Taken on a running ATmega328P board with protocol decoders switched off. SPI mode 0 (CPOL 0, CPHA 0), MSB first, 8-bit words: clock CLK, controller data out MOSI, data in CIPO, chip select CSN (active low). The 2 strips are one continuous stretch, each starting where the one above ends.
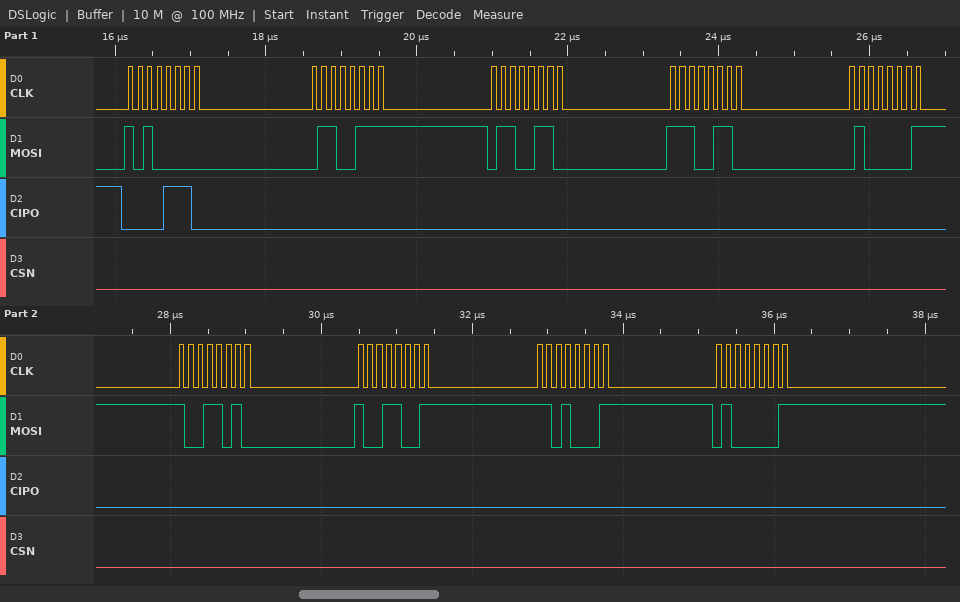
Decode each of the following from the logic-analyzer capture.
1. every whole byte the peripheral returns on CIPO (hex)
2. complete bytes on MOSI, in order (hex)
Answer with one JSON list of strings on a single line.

["0E 00 00 00 00 00 00 00 00", "A0 67 66 E6 41 9A 99 D1 41"]
